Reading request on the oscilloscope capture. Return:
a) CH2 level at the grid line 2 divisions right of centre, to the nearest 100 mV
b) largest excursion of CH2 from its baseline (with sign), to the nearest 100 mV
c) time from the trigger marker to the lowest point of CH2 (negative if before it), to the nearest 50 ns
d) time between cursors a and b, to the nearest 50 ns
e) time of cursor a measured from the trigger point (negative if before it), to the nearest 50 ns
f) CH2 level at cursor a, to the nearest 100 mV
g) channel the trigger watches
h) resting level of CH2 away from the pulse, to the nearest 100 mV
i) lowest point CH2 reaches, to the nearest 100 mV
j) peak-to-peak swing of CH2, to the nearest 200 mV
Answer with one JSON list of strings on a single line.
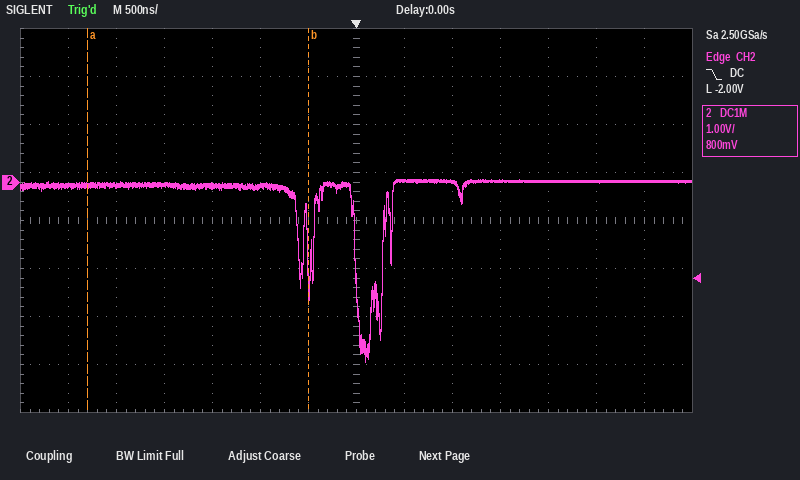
["0.0 V", "-3.7 V", "+100 ns", "2.30 µs", "-2.80 µs", "-100 mV", "CH2", "0.0 V", "-3.7 V", "3.8 V"]
